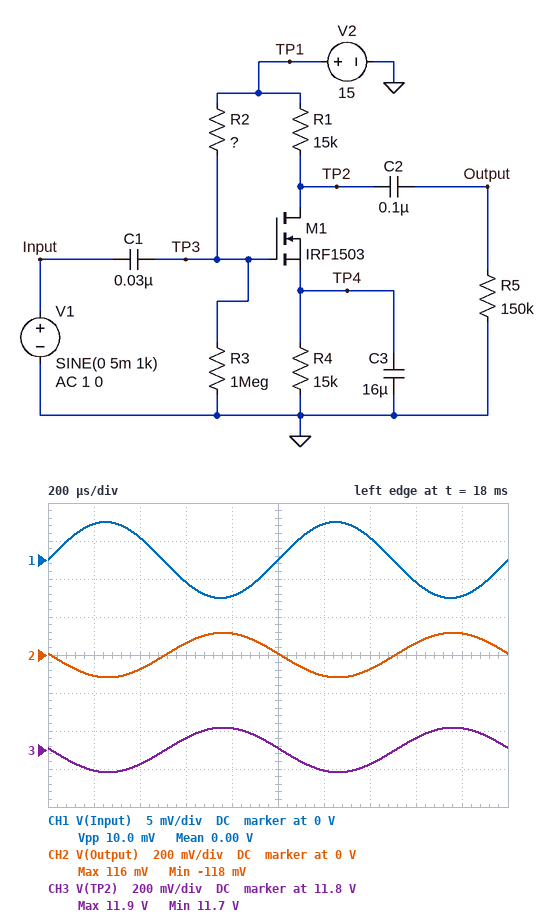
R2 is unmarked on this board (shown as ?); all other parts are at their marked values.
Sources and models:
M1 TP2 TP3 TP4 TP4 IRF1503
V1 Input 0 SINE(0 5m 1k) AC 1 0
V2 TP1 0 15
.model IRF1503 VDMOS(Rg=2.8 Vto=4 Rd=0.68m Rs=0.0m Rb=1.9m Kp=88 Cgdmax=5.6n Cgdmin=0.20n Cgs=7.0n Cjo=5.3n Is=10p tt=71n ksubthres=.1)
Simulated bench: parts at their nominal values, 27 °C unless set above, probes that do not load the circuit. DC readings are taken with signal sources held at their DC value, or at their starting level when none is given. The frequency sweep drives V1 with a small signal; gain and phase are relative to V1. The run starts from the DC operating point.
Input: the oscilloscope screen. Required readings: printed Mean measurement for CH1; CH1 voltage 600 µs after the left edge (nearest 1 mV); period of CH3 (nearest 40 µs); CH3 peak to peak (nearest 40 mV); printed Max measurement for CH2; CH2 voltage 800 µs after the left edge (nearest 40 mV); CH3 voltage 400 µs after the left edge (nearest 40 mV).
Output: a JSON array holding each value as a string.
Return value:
["0.00 V", "-3 mV", "1.00 ms", "240 mV", "116 mV", "120 mV", "11.72 V"]
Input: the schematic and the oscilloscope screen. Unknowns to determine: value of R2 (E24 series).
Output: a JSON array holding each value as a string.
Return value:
["1.2 MΩ"]
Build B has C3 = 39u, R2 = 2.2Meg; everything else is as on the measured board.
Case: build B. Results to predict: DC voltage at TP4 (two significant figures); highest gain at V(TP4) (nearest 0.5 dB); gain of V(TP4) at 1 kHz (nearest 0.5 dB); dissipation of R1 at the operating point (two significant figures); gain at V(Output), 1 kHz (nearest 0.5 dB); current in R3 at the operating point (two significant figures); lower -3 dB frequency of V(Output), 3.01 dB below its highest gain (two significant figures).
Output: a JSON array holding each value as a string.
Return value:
["1.1 V", "-7.5 dB", "-48.0 dB", "84 µW", "22.5 dB", "4.7 µA", "12 Hz"]
